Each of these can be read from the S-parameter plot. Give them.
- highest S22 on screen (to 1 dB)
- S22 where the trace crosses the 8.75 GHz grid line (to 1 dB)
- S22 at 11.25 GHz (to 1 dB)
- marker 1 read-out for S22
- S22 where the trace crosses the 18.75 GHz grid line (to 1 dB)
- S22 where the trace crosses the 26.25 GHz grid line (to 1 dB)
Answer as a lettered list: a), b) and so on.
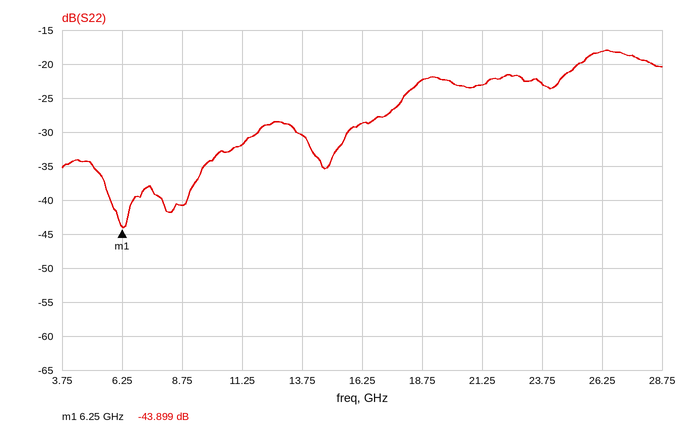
a) -18 dB
b) -41 dB
c) -32 dB
d) -43.899 dB
e) -22 dB
f) -18 dB
